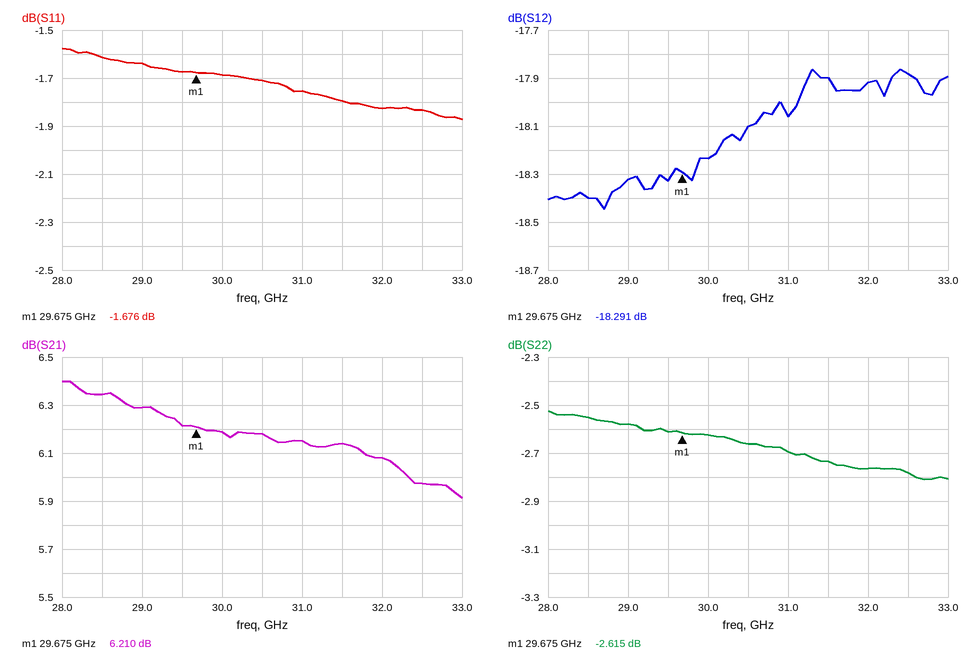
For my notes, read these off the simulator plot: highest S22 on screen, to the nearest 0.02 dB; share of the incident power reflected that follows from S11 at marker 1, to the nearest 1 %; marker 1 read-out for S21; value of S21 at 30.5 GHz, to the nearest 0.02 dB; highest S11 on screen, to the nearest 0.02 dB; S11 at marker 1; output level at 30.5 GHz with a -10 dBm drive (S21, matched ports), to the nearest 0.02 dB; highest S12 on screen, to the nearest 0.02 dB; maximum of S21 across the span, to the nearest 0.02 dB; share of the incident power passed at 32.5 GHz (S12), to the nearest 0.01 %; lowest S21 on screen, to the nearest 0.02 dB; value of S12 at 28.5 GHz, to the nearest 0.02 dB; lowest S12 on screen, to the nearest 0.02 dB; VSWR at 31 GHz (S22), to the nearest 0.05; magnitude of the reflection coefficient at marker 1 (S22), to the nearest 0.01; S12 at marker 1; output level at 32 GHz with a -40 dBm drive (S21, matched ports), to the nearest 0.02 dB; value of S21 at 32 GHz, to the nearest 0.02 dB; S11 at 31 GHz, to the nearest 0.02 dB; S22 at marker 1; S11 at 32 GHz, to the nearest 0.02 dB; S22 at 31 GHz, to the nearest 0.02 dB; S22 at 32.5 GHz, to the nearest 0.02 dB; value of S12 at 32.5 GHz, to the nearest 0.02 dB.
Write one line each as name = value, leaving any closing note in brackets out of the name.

highest S22 on screen, to the nearest 0.02 dB = -2.52 dB
share of the incident power reflected that follows from S11 at marker 1, to the nearest 1 % = 68 %
marker 1 read-out for S21 = 6.210 dB
value of S21 at 30.5 GHz, to the nearest 0.02 dB = 6.18 dB
highest S11 on screen, to the nearest 0.02 dB = -1.58 dB
S11 at marker 1 = -1.676 dB
output level at 30.5 GHz with a -10 dBm drive (S21, matched ports), to the nearest 0.02 dB = -3.82 dBm
highest S12 on screen, to the nearest 0.02 dB = -17.86 dB
maximum of S21 across the span, to the nearest 0.02 dB = 6.40 dB
share of the incident power passed at 32.5 GHz (S12), to the nearest 0.01 % = 1.63 %
lowest S21 on screen, to the nearest 0.02 dB = 5.92 dB
value of S12 at 28.5 GHz, to the nearest 0.02 dB = -18.40 dB
lowest S12 on screen, to the nearest 0.02 dB = -18.44 dB
VSWR at 31 GHz (S22), to the nearest 0.05 = 6.50
magnitude of the reflection coefficient at marker 1 (S22), to the nearest 0.01 = 0.74
S12 at marker 1 = -18.291 dB
output level at 32 GHz with a -40 dBm drive (S21, matched ports), to the nearest 0.02 dB = -33.92 dBm
value of S21 at 32 GHz, to the nearest 0.02 dB = 6.08 dB
S11 at 31 GHz, to the nearest 0.02 dB = -1.76 dB
S22 at marker 1 = -2.615 dB
S11 at 32 GHz, to the nearest 0.02 dB = -1.82 dB
S22 at 31 GHz, to the nearest 0.02 dB = -2.70 dB
S22 at 32.5 GHz, to the nearest 0.02 dB = -2.78 dB
value of S12 at 32.5 GHz, to the nearest 0.02 dB = -17.88 dB
